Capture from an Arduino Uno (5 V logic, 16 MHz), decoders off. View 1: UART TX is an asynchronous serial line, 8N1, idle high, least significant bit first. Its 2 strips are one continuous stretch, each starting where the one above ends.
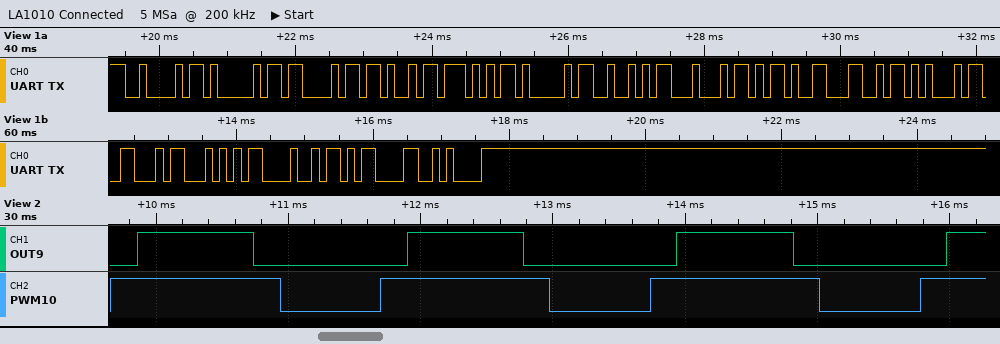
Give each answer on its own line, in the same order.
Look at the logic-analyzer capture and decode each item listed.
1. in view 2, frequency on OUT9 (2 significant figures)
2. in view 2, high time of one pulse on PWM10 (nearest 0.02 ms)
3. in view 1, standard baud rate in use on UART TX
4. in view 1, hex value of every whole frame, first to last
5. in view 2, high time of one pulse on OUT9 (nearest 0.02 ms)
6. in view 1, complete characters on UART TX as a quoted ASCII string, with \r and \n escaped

490 Hz
1.28 ms
9600 baud
0x42 0x41 0x43 0x4B 0x57 0x41 0x52 0x44 0x2D 0x4C 0x45 0x46 0x54 0x48 0x0D 0x0A
0.88 ms
"BACKWARD-LEFTH\r\n"
